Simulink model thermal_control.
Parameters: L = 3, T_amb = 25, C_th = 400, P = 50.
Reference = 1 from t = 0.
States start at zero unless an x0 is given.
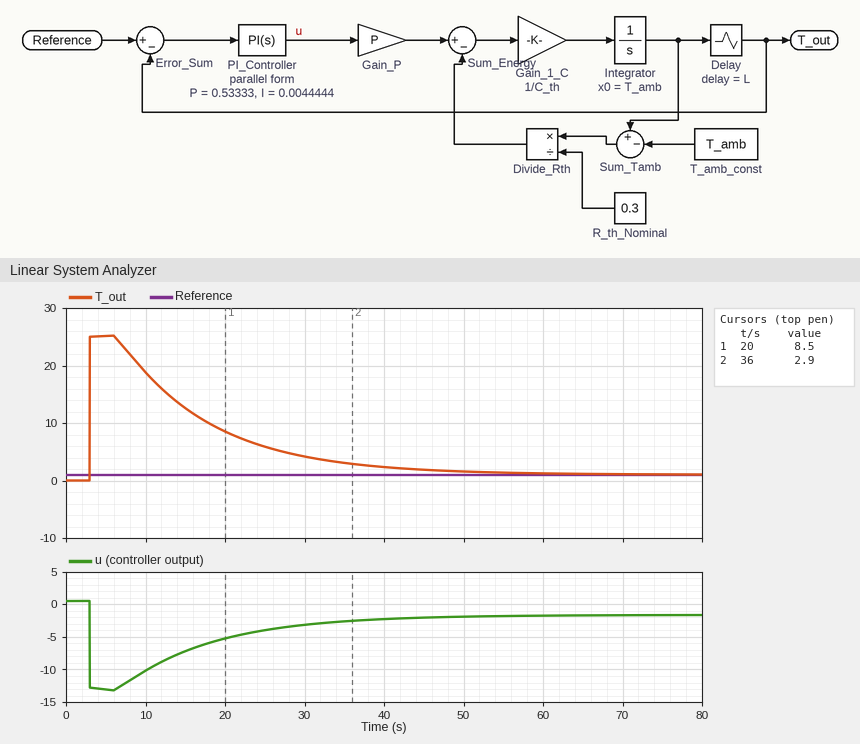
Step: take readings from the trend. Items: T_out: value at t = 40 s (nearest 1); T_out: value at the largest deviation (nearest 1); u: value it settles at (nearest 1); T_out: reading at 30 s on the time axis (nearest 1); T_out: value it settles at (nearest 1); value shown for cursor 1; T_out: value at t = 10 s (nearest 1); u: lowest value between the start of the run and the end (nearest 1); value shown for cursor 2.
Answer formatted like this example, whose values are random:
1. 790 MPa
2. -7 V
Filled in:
1. 2
2. 25
3. -2
4. 4
5. 1
6. 8.5
7. 19
8. -13
9. 2.9
